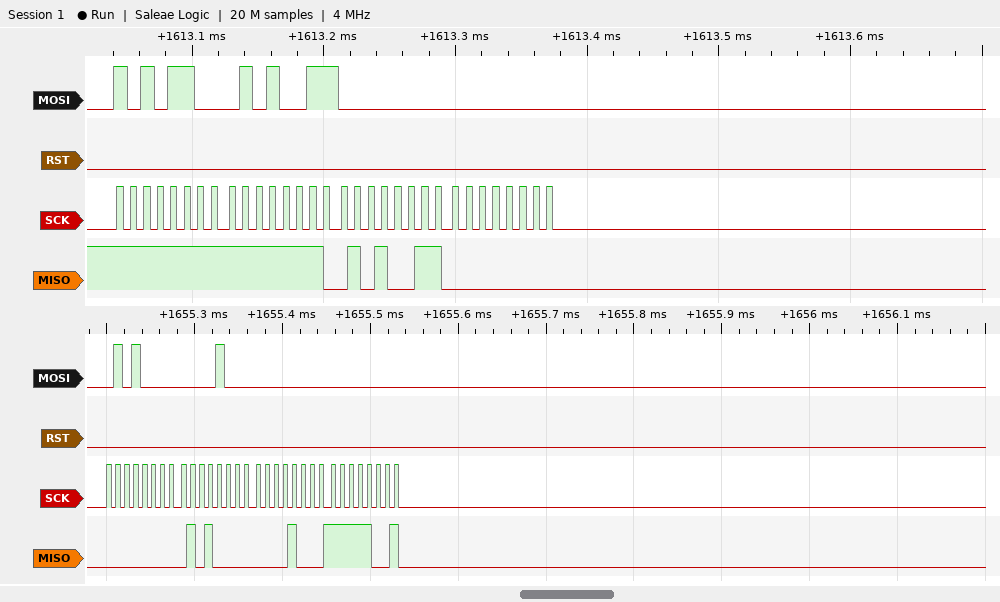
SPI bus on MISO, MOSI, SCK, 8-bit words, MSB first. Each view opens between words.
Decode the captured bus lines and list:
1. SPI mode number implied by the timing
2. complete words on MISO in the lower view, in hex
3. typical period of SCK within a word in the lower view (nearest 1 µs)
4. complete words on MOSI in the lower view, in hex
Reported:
0
00, 50, 08, F9
10 µs
50, 08, 00, 00
